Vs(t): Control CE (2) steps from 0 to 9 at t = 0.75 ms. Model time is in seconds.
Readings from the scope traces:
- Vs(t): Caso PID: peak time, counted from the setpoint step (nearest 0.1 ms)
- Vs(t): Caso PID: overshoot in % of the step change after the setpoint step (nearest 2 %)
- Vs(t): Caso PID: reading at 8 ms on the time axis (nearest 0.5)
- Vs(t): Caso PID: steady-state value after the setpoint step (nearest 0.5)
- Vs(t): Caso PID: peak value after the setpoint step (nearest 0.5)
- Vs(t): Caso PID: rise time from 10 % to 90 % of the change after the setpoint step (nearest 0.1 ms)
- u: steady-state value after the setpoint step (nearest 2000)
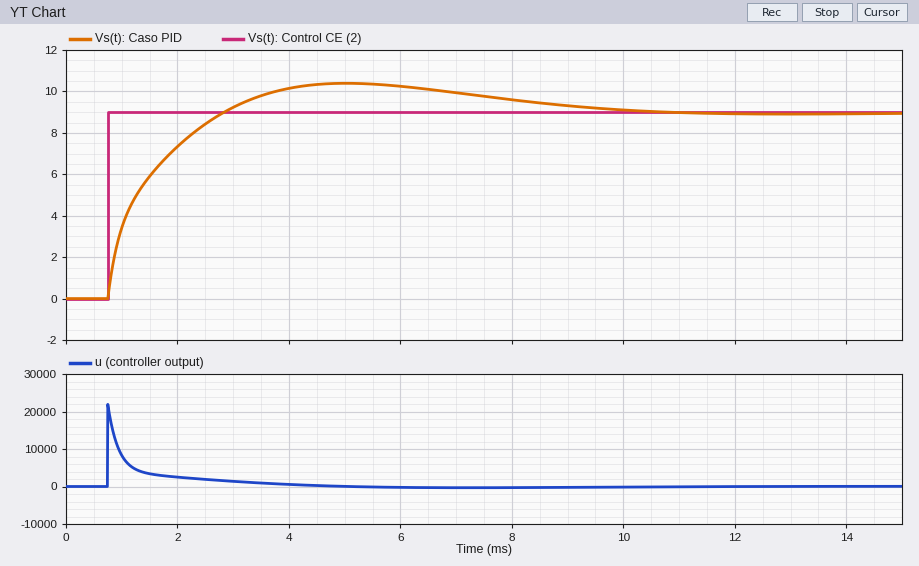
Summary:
4.3 ms
16 %
9.5
9.0
10.5
1.5 ms
0
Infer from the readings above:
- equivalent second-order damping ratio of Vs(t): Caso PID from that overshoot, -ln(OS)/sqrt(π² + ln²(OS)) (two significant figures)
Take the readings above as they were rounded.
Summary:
0.50
